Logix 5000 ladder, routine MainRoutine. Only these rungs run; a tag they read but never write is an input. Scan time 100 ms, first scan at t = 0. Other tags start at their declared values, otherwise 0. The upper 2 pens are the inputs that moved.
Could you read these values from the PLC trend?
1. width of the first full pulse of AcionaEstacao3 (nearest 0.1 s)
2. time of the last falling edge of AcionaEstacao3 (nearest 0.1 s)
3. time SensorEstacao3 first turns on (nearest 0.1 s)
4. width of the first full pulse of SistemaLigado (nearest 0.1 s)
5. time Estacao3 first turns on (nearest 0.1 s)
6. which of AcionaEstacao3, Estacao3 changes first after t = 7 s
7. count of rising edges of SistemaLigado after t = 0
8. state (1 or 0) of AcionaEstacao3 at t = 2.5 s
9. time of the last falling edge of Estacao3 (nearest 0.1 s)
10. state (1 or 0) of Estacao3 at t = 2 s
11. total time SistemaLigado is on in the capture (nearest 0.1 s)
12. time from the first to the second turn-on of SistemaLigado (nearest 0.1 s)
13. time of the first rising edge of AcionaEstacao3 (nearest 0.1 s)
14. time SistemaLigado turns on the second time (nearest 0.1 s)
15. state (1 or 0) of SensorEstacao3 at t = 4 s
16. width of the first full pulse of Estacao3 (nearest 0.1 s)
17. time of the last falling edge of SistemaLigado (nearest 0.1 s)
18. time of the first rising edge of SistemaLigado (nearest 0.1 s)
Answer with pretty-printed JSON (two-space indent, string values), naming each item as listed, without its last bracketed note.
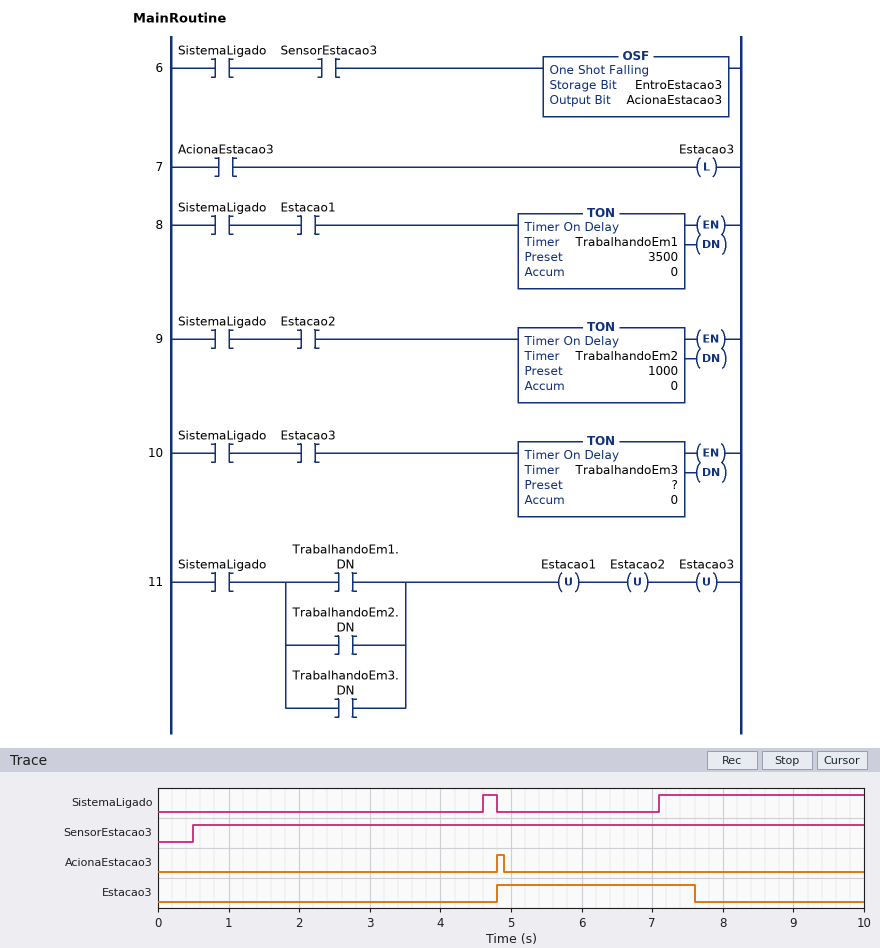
{
  "width of the first full pulse of AcionaEstacao3": "0.1 s",
  "time of the last falling edge of AcionaEstacao3": "4.9 s",
  "time SensorEstacao3 first turns on": "0.5 s",
  "width of the first full pulse of SistemaLigado": "0.2 s",
  "time Estacao3 first turns on": "4.8 s",
  "which of AcionaEstacao3, Estacao3 changes first after t = 7 s": "Estacao3",
  "count of rising edges of SistemaLigado after t = 0": "2",
  "state (1 or 0) of AcionaEstacao3 at t = 2.5 s": "0",
  "time of the last falling edge of Estacao3": "7.6 s",
  "state (1 or 0) of Estacao3 at t = 2 s": "0",
  "total time SistemaLigado is on in the capture": "3.1 s",
  "time from the first to the second turn-on of SistemaLigado": "2.5 s",
  "time of the first rising edge of AcionaEstacao3": "4.8 s",
  "time SistemaLigado turns on the second time": "7.1 s",
  "state (1 or 0) of SensorEstacao3 at t = 4 s": "1",
  "width of the first full pulse of Estacao3": "2.8 s",
  "time of the last falling edge of SistemaLigado": "4.8 s",
  "time of the first rising edge of SistemaLigado": "4.6 s"
}
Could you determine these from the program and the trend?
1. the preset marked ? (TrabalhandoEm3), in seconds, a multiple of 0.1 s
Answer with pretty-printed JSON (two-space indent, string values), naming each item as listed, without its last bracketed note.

{
  "the preset marked ? (TrabalhandoEm3), in seconds, a multiple of 0.1 s": "0.5 s"
}
